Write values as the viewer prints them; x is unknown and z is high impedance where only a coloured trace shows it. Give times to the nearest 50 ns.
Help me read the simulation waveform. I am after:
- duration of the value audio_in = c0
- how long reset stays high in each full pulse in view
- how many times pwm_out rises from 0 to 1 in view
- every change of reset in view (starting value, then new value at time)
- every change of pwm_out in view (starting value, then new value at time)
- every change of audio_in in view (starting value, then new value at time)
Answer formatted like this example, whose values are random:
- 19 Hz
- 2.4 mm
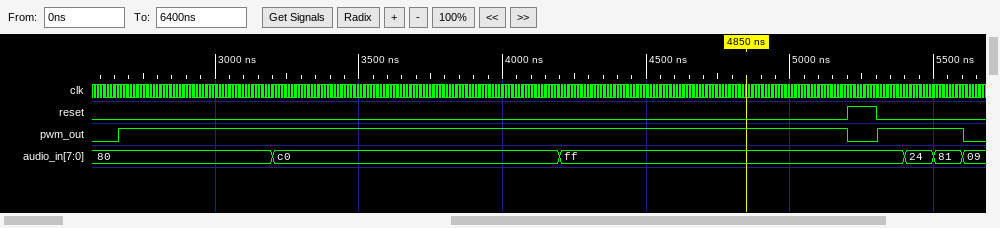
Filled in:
- 1000 ns
- 100 ns
- 2
- 0, 1 at 5200 ns, 0 at 5300 ns
- 0, 1 at 2650 ns, 0 at 5200 ns, 1 at 5300 ns, 0 at 5600 ns
- 80, c0 at 3200 ns, ff at 4200 ns, 24 at 5400 ns, 81 at 5500 ns, 09 at 5600 ns
